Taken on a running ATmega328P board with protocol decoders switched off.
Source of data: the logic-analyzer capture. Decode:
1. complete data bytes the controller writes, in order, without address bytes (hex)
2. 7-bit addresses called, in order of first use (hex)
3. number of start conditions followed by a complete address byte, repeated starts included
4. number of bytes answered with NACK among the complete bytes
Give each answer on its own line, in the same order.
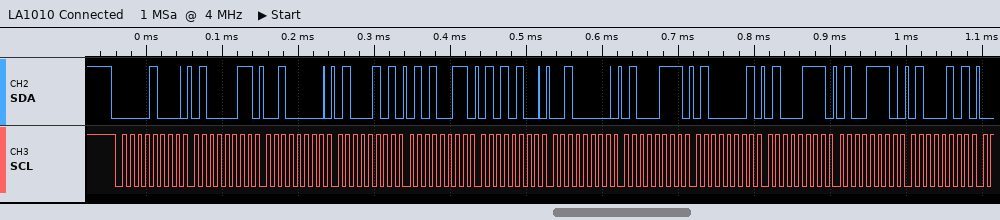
43 20 45 53 54 20 47 41 47 4E 45
0x04
1
0
